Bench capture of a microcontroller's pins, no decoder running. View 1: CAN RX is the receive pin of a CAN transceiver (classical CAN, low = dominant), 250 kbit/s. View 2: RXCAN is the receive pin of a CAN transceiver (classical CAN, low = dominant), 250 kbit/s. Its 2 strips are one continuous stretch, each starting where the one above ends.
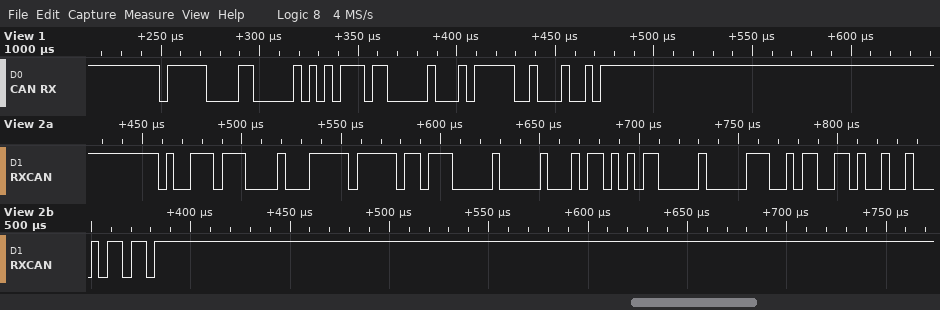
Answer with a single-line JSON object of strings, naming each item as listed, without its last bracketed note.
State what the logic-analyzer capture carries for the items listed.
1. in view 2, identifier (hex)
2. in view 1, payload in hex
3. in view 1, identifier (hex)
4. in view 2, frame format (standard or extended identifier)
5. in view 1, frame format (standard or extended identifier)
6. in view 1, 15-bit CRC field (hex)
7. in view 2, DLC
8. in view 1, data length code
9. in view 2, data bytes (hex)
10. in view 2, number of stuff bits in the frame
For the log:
{"in view 2, identifier": "0x4EE", "in view 1, payload in hex": "BB 00", "in view 1, identifier": "0x7C6", "in view 2, frame format": "standard", "in view 1, frame format": "standard", "in view 1, 15-bit CRC field": "0x5F44", "in view 2, DLC": "8", "in view 1, data length code": "2", "in view 2, data bytes": "FF F7 00 05 AB 00 32 CD", "in view 2, number of stuff bits in the frame": "6"}
